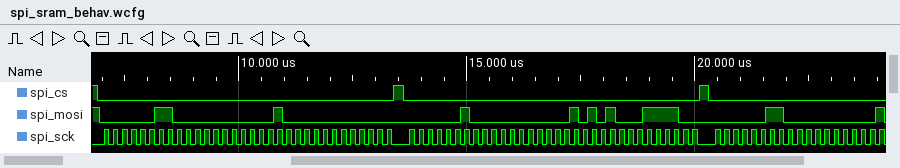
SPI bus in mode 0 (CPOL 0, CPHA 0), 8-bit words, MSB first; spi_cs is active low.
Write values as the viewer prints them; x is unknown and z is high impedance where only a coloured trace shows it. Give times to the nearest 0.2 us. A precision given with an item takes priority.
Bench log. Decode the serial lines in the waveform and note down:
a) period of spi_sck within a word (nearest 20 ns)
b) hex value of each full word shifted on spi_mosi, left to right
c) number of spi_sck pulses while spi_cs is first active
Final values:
200 ns
03, 00, 10, 00, 02, 00, 2A, 3C, 03, 00
32
